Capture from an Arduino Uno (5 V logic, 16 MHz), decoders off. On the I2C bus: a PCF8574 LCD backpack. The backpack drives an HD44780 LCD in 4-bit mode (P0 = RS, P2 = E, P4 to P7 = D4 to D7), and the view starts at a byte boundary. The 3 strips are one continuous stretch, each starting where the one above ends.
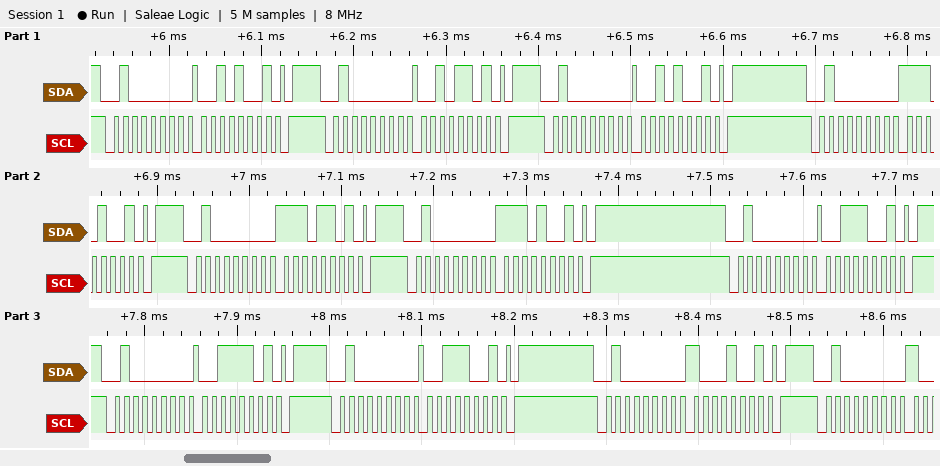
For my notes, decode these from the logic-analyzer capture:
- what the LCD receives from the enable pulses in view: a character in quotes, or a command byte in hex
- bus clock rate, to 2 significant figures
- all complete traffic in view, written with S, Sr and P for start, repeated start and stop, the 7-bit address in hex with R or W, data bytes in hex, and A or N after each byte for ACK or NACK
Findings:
'.'
100 kHz
S 20W A 29 A P S 20W A 2D A P S 20W A 29 A P S 20W A E9 A P S 20W A ED A P S 20W A E9 A P S 20W A 39 A P S 20W A 3D A P S 20W A 39 A P S 20W A 89 A P S 20W A
